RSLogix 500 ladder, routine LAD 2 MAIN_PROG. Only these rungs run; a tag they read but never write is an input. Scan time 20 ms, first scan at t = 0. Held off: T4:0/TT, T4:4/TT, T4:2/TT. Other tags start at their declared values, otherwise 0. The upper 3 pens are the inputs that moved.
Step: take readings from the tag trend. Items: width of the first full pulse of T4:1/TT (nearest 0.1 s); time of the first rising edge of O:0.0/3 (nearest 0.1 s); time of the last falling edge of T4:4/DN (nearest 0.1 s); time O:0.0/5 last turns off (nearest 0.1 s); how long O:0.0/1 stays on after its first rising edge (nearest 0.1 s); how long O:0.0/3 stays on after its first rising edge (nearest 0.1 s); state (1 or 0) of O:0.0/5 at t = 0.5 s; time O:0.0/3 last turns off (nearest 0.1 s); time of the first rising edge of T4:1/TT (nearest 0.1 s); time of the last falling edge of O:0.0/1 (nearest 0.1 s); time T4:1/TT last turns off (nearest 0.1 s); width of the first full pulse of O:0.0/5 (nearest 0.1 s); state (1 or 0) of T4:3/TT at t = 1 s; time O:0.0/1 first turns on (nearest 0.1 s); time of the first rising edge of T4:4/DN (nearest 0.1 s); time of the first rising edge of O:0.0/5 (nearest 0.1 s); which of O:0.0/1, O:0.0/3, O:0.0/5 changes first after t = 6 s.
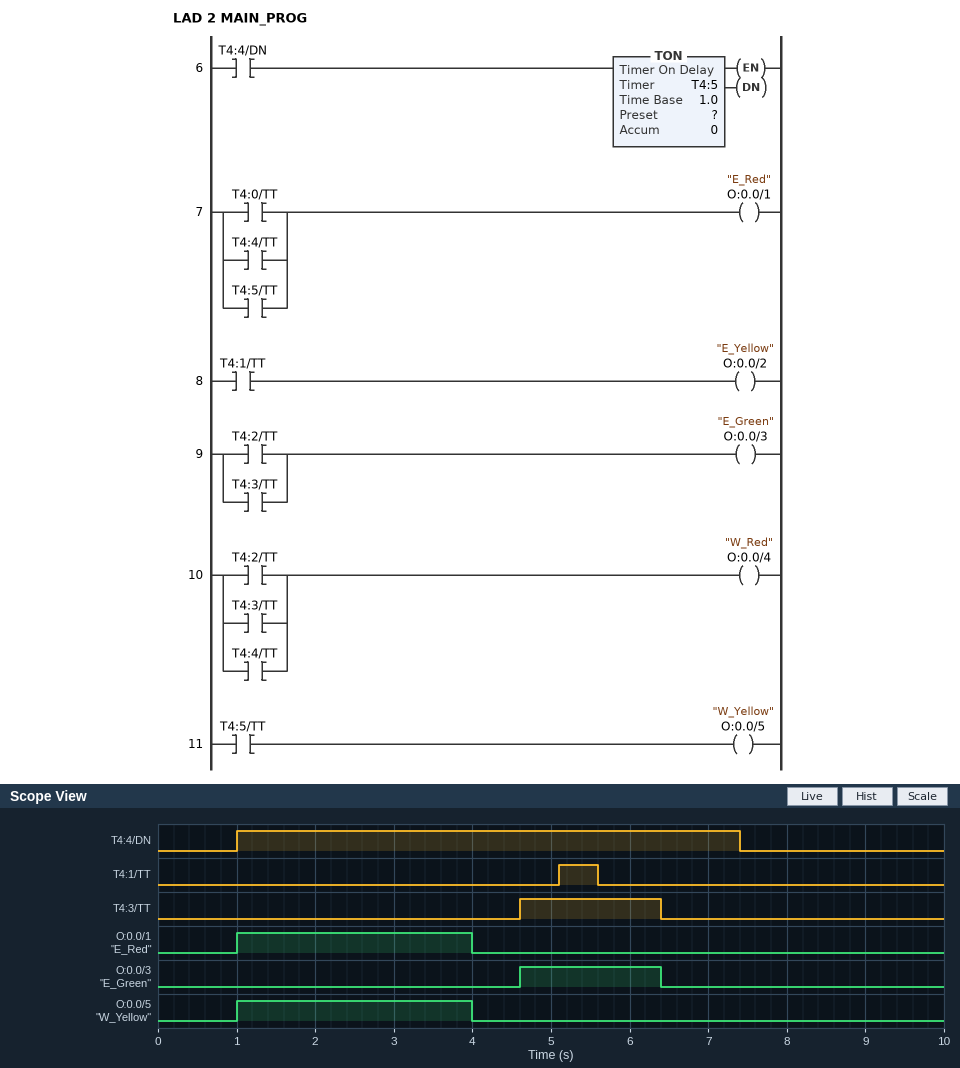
0.5 s
4.6 s
7.4 s
4.0 s
3.0 s
1.8 s
0
6.4 s
5.1 s
4.0 s
5.6 s
3.0 s
0
1.0 s
1.0 s
1.0 s
O:0.0/3
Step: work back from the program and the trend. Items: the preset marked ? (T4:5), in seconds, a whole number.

3 s
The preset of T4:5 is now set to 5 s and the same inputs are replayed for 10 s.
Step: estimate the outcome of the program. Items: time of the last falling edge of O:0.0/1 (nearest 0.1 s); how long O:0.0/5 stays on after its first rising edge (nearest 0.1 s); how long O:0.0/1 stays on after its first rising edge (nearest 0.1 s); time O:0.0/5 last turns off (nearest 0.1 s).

6.0 s
5.0 s
5.0 s
6.0 s
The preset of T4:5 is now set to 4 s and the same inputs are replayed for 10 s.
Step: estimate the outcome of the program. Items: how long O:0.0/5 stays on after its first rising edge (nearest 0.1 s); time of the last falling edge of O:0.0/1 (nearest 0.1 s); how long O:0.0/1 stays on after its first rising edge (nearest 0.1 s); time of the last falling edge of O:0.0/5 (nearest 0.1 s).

4.0 s
5.0 s
4.0 s
5.0 s
